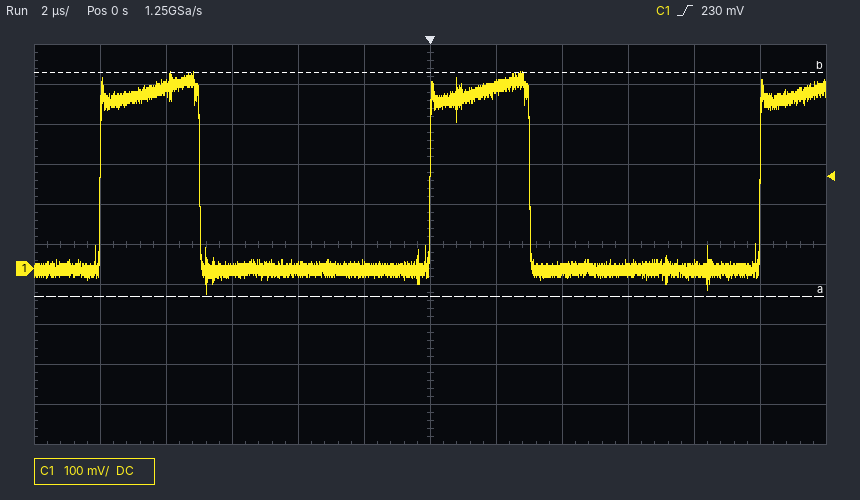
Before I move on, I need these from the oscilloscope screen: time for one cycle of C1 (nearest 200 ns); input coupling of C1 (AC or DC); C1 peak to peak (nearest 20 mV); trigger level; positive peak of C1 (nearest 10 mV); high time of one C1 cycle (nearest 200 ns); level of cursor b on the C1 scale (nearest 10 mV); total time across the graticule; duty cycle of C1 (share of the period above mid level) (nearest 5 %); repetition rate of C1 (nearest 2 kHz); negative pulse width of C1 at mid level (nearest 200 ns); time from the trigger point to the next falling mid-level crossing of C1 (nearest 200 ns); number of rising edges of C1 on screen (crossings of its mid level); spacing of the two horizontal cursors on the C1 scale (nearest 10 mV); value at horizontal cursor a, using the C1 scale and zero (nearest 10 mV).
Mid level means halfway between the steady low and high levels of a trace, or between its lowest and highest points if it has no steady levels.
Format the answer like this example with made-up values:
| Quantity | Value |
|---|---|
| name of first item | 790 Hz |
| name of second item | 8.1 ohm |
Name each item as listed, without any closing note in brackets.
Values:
| Quantity | Value |
|---|---|
| time for one cycle of C1 | 10.0 µs |
| input coupling of C1 | DC |
| C1 peak to peak | 560 mV |
| trigger level | 230 mV |
| positive peak of C1 | 490 mV |
| high time of one C1 cycle | 3.0 µs |
| level of cursor b on the C1 scale | 490 mV |
| total time across the graticule | 24 µs |
| duty cycle of C1 (share of the period above mid level) | 30 % |
| repetition rate of C1 | 100 kHz |
| negative pulse width of C1 at mid level | 7.0 µs |
| time from the trigger point to the next falling mid-level crossing of C1 | 3.0 µs |
| number of rising edges of C1 on screen | 3 |
| spacing of the two horizontal cursors on the C1 scale | 560 mV |
| value at horizontal cursor a, using the C1 scale and zero | -70 mV |
